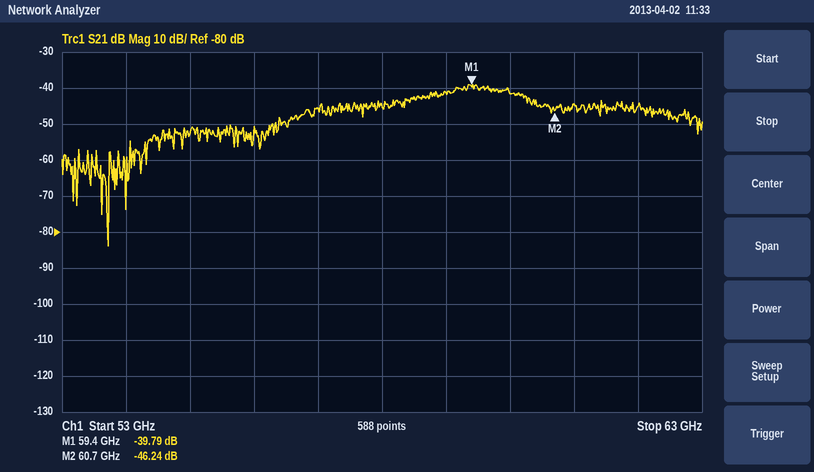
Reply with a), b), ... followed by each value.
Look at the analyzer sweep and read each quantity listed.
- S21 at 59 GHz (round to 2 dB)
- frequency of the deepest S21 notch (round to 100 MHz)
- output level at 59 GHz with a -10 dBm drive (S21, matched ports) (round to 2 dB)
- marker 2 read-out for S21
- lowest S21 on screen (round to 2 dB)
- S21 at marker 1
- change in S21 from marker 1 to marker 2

a) -42 dB
b) 53.7 GHz
c) -52 dBm
d) -46.24 dB
e) -84 dB
f) -39.79 dB
g) -6.45 dB
